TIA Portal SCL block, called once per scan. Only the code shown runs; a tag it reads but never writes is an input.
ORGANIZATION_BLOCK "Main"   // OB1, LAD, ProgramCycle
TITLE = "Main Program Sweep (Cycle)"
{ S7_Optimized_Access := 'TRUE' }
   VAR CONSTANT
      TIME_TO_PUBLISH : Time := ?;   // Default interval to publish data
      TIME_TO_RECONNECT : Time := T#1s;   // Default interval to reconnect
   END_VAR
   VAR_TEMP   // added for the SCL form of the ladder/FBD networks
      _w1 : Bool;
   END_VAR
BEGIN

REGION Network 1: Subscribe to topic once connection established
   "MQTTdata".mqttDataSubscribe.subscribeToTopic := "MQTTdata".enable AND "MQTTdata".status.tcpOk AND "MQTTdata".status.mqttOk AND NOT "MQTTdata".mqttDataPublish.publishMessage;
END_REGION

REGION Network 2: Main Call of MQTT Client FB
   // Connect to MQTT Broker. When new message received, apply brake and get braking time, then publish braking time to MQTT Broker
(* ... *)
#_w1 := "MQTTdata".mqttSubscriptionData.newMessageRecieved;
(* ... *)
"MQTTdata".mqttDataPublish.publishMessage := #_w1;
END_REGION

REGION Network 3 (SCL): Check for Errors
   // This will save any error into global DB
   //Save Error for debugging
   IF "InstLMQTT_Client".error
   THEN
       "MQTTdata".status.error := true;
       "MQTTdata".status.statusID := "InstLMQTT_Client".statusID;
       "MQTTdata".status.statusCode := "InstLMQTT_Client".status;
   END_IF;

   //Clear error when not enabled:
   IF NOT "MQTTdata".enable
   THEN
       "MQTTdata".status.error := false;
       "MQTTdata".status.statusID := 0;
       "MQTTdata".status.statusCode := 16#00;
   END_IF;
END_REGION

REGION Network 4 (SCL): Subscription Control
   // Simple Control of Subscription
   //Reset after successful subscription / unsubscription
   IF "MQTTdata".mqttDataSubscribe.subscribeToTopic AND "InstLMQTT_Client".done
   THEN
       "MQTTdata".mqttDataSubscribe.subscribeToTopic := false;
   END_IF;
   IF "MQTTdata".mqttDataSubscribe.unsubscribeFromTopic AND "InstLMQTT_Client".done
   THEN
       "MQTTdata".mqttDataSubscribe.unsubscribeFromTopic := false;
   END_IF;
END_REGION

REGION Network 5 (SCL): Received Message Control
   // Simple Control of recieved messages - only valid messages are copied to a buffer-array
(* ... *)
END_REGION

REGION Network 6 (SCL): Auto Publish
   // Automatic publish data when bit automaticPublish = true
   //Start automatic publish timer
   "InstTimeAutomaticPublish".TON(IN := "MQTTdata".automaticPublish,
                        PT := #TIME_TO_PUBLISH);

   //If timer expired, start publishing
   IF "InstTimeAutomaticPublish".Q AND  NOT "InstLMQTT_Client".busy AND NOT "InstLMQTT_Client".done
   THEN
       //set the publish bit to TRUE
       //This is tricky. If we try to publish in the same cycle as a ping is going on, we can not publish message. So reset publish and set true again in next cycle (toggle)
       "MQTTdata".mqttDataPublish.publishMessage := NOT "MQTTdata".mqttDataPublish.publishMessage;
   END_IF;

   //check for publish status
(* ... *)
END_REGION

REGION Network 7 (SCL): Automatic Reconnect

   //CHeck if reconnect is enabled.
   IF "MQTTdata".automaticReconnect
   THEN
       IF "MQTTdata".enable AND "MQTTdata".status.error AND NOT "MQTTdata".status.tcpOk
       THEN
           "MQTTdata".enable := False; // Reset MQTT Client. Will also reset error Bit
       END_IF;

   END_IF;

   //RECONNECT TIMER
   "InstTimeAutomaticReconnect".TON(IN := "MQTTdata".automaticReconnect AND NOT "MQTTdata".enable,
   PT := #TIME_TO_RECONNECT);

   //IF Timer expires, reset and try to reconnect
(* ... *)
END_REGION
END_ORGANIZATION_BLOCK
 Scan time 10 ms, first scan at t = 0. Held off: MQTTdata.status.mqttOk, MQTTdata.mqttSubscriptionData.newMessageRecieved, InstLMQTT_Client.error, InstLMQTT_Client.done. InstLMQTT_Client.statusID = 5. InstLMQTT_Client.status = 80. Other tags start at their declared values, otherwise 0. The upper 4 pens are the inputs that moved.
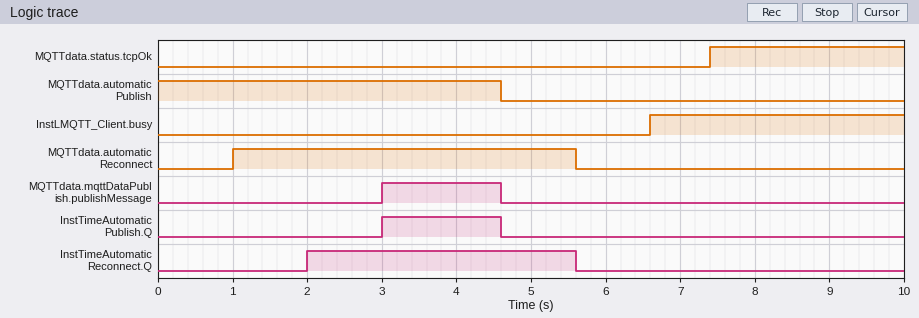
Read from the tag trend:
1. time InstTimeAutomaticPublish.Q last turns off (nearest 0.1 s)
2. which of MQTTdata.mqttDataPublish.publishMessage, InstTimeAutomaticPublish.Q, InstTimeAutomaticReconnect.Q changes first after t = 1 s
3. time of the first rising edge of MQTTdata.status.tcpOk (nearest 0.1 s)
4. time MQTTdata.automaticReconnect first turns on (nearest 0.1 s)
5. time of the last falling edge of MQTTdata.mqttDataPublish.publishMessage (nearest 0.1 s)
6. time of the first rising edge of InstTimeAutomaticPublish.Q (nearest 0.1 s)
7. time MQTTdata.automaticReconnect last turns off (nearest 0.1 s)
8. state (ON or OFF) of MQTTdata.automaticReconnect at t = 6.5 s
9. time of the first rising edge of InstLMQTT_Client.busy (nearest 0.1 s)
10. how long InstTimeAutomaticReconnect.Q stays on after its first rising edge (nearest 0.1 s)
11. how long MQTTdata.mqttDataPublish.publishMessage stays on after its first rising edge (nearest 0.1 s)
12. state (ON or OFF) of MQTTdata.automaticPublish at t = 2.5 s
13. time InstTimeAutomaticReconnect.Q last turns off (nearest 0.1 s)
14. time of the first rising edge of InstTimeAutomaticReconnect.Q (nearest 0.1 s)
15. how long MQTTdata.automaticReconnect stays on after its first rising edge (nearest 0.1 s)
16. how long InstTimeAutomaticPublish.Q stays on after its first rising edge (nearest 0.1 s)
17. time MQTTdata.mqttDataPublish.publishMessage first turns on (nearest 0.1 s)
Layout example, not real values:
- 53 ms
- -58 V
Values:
- 4.6 s
- InstTimeAutomaticReconnect.Q
- 7.4 s
- 1.0 s
- 4.6 s
- 3.0 s
- 5.6 s
- OFF
- 6.6 s
- 3.6 s
- 1.6 s
- ON
- 5.6 s
- 2.0 s
- 4.6 s
- 1.6 s
- 3.0 s
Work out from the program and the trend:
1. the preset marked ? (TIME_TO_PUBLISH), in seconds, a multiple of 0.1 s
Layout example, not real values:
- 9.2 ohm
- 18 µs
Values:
- 3.0 s
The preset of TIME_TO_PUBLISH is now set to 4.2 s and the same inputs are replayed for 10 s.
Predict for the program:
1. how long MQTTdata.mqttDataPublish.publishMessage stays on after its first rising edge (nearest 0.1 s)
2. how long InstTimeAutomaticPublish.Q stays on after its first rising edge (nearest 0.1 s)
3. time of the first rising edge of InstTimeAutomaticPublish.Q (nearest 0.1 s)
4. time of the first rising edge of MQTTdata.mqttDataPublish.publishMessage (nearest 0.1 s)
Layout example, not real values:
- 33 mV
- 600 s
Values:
- 0.4 s
- 0.4 s
- 4.2 s
- 4.2 s
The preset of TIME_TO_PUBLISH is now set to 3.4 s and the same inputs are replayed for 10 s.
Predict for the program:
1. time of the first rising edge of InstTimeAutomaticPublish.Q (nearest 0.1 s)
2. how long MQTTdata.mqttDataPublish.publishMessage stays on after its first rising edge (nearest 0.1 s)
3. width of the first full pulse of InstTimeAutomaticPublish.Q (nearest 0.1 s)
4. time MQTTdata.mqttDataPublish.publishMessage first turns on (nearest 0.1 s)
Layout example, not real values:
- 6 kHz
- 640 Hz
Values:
- 3.4 s
- 1.2 s
- 1.2 s
- 3.4 s
